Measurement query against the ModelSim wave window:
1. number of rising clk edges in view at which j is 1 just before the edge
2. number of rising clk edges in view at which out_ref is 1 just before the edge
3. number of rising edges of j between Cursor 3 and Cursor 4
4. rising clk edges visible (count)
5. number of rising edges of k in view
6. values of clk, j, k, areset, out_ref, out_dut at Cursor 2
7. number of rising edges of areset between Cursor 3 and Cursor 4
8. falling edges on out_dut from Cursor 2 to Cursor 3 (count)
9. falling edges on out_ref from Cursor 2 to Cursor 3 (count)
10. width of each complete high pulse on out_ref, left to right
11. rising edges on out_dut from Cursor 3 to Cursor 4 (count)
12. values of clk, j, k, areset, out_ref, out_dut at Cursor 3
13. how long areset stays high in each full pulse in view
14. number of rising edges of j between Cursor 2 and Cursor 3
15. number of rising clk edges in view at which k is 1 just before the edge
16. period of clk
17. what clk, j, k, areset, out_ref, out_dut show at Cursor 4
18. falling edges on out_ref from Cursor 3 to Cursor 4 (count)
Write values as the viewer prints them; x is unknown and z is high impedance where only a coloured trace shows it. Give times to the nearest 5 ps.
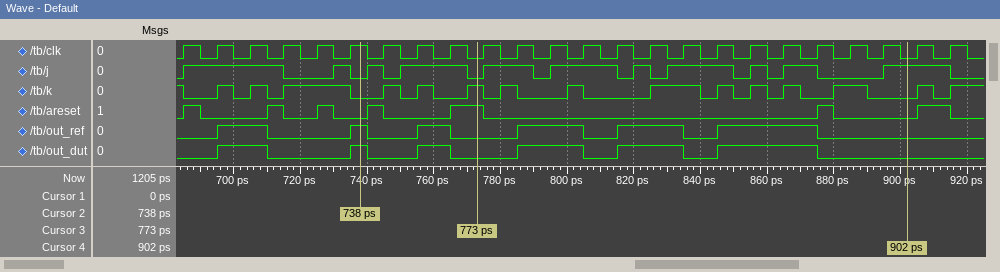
16
9
7
24
15
clk=1, j=0, k=0, areset=0, out_ref=1, out_dut=1
1
2
2
15 ps, 5 ps, 10 ps, 20 ps, 20 ps, 30 ps
3
clk=0, j=0, k=1, areset=1, out_ref=0, out_dut=0
5 ps, 5 ps, 5 ps, 5 ps, 10 ps, 5 ps, 10 ps
2
8
10 ps
clk=0, j=1, k=0, areset=0, out_ref=0, out_dut=0
3
